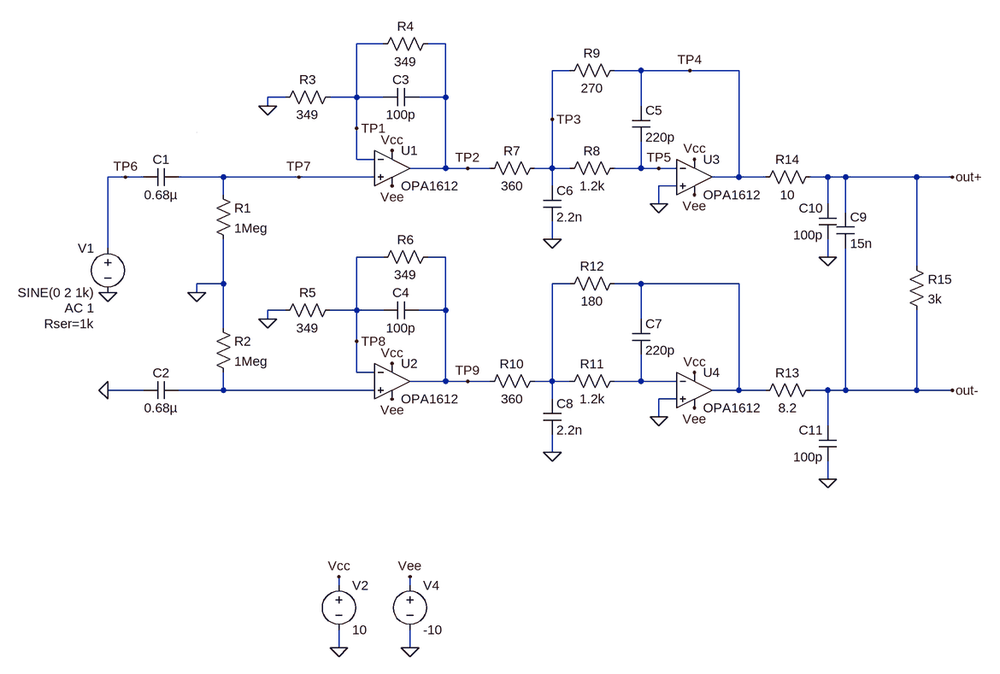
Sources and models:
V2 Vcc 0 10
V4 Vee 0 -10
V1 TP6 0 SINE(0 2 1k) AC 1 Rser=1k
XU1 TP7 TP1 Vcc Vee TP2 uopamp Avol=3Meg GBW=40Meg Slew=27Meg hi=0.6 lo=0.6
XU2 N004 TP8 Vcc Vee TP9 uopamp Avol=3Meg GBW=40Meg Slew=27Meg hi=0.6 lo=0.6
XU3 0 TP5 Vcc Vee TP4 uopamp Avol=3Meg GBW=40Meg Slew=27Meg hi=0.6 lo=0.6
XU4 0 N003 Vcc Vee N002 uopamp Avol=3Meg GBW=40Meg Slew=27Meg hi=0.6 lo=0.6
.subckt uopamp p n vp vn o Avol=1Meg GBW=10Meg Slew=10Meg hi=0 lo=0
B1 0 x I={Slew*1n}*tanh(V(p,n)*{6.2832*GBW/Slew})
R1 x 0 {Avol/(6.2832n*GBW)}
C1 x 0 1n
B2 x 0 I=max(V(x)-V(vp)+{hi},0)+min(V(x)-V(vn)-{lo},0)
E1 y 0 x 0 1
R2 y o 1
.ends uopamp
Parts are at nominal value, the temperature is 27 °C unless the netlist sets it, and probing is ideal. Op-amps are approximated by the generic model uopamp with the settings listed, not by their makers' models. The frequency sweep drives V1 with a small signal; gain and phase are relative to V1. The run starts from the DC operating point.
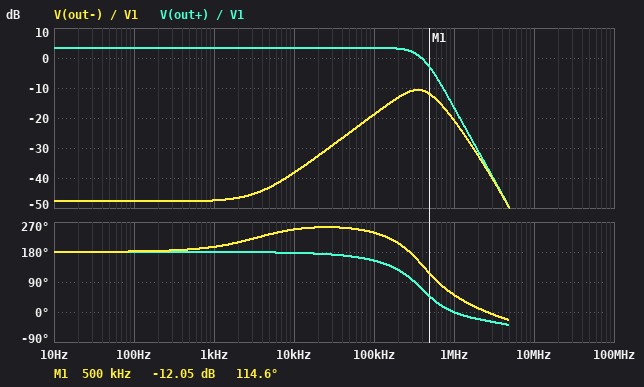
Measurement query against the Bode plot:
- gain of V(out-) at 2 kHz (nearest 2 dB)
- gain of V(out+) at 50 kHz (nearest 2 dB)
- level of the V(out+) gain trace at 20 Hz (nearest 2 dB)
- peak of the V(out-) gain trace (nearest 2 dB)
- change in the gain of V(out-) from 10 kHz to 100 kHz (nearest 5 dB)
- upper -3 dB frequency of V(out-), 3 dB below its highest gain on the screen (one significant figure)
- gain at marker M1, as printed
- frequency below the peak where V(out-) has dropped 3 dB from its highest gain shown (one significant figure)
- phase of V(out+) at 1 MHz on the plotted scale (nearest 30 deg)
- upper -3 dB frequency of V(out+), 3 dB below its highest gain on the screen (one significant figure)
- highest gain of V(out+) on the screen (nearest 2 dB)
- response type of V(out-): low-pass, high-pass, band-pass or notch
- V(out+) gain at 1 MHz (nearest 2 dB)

-46 dB
4 dB
4 dB
-10 dB
20 dB
600 kHz
-12.05 dB
200 kHz
0 deg
400 kHz
4 dB
band-pass
-16 dB
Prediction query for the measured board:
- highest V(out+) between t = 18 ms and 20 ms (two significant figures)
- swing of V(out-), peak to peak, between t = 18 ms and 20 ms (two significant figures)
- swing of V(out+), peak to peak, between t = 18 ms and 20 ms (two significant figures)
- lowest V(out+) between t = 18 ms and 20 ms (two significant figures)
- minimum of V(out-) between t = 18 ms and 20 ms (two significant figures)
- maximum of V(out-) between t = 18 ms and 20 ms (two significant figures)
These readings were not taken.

3.0 V
17 mV
6.0 V
-3.0 V
-8.5 mV
8.5 mV
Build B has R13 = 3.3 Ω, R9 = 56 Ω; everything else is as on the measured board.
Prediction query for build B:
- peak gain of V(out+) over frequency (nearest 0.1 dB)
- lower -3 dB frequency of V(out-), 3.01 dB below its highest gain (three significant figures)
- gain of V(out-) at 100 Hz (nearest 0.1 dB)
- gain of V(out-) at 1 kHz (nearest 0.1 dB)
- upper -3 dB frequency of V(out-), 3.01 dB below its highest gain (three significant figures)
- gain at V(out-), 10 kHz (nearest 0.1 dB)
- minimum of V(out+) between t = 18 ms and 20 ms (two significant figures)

-10.2 dB
293 kHz
-69.4 dB
-69.0 dB
1.18 MHz
-59.8 dB
-620 mV
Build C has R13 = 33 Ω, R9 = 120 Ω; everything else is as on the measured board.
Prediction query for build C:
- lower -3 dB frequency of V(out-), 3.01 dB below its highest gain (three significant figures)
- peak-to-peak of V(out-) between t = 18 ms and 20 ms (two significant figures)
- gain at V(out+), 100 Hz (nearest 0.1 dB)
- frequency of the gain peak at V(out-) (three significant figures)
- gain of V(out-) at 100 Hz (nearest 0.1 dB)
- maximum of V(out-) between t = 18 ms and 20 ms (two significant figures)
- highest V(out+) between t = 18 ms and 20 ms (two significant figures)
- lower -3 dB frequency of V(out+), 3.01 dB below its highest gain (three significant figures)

162 kHz
30 mV
-3.6 dB
381 kHz
-42.8 dB
15 mV
1.3 V
234 mHz
